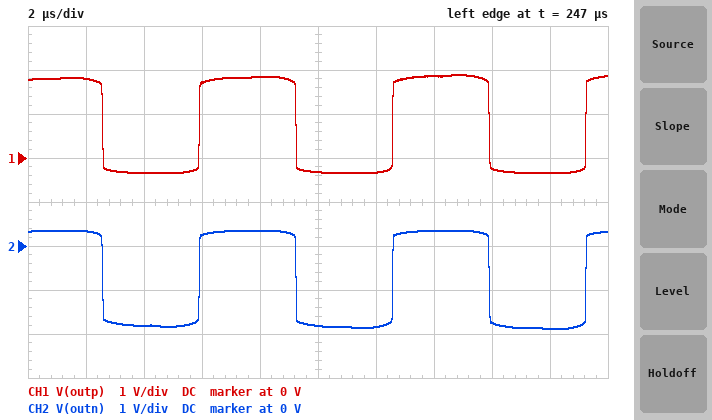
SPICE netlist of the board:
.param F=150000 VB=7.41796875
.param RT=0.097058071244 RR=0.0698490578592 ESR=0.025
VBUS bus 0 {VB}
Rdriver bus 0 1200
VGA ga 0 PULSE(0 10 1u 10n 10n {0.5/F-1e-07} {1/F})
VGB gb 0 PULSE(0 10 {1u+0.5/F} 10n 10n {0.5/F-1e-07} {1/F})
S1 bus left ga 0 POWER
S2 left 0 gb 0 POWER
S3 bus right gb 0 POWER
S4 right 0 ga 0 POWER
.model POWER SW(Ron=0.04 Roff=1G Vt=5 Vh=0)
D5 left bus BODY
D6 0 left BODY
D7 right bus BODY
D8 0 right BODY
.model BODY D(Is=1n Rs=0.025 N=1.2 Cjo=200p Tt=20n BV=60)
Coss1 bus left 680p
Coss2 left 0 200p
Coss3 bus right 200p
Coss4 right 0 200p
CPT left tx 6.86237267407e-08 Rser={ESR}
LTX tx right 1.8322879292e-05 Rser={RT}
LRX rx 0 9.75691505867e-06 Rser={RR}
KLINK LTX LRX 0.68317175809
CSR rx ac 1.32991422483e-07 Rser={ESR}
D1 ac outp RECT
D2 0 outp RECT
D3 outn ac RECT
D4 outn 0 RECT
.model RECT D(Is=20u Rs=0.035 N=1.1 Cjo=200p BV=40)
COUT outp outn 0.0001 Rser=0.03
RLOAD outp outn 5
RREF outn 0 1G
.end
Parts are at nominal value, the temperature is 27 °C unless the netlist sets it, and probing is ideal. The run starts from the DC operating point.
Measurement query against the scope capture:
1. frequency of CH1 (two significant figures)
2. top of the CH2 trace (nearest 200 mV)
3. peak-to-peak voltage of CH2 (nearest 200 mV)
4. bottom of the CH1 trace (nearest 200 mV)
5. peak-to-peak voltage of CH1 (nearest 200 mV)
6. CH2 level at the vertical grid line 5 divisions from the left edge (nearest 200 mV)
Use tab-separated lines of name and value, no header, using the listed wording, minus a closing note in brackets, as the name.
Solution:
frequency of CH1	150 kHz
top of the CH2 trace	400 mV
peak-to-peak voltage of CH2	2.2 V
bottom of the CH1 trace	-400 mV
peak-to-peak voltage of CH1	2.2 V
CH2 level at the vertical grid line 5 divisions from the left edge	-1.8 V
